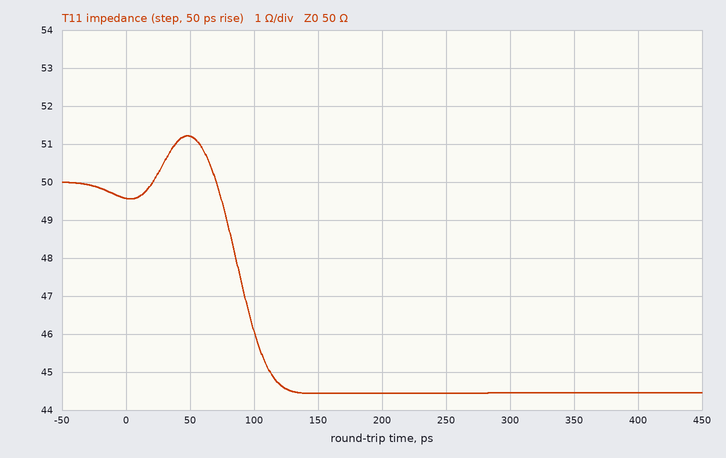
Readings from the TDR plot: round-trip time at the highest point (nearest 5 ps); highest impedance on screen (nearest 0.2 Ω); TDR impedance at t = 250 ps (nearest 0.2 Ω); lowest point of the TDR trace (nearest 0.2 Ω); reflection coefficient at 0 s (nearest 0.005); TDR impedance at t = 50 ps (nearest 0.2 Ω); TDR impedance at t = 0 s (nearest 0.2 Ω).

50 ps
51.2 Ω
44.4 Ω
44.4 Ω
-0.005
51.2 Ω
49.6 Ω
